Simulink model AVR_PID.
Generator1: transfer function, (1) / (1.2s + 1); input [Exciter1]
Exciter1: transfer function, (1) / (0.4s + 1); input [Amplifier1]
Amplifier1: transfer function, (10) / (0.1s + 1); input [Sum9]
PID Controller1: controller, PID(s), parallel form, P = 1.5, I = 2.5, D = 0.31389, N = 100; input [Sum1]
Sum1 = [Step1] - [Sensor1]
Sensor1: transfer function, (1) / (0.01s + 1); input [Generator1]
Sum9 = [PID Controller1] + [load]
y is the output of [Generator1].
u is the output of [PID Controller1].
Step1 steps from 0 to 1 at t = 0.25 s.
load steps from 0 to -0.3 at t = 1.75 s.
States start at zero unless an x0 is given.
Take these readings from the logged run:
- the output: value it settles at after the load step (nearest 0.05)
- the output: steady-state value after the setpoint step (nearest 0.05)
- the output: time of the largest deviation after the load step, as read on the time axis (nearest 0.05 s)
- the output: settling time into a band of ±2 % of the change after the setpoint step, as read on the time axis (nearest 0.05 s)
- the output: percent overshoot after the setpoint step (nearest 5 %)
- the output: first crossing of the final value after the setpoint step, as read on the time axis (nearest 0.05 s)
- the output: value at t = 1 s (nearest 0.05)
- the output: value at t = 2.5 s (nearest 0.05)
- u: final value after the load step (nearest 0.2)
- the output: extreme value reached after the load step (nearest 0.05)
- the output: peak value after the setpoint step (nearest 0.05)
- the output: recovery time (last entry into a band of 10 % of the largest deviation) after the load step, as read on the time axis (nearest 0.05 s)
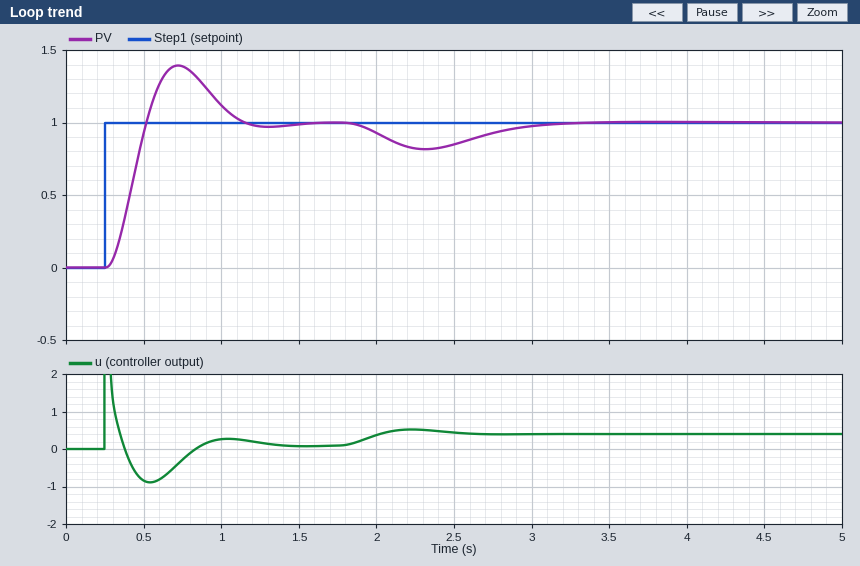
1.00
1.00
2.30 s
1.45 s
40 %
0.50 s
1.10
0.85
0.4
0.80
1.40
3.05 s
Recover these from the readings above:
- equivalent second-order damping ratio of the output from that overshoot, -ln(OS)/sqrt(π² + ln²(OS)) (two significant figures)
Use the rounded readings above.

0.28
